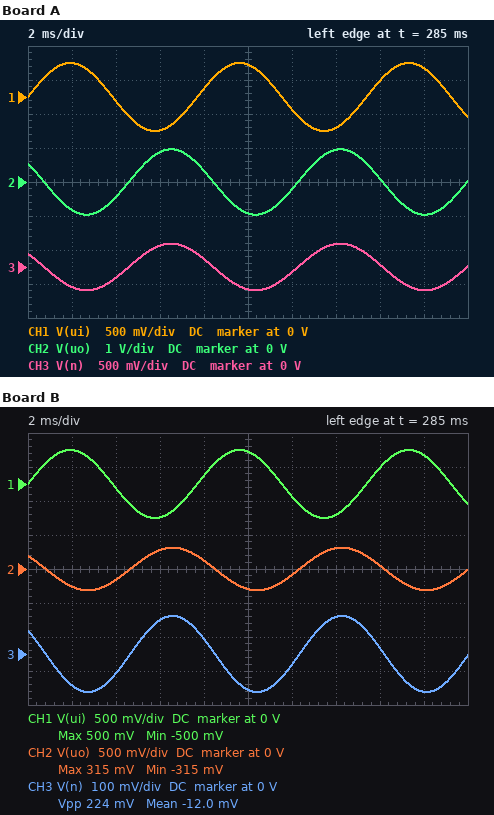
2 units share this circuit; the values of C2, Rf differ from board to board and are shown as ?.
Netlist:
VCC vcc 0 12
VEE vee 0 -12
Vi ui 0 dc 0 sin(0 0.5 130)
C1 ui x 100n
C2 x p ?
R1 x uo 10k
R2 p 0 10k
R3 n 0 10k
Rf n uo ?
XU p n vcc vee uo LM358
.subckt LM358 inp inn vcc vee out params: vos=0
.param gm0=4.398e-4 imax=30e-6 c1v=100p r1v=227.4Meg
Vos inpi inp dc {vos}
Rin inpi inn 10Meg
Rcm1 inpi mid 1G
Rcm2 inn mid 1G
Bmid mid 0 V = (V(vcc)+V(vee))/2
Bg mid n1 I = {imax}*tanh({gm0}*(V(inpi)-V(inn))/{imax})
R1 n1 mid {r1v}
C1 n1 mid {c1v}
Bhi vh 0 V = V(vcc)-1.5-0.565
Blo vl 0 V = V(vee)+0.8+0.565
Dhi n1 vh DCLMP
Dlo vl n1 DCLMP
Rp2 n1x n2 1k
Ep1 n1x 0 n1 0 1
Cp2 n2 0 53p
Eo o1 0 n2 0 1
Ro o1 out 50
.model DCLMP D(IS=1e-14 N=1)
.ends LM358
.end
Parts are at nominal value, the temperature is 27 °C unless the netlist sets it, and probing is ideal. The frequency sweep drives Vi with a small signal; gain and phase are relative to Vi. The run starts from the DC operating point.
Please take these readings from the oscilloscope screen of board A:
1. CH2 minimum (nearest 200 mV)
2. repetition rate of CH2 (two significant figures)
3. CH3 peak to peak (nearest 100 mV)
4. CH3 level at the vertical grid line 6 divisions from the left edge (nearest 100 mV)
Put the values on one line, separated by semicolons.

-1.0 V; 130 Hz; 700 mV; -100 mV
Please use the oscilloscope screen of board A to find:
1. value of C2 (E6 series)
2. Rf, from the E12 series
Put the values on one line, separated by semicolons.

68 nF; 18 kΩ
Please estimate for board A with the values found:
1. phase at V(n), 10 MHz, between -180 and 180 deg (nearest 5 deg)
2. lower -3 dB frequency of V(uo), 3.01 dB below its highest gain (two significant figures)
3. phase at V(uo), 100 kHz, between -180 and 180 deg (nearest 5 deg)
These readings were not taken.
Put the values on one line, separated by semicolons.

-155 deg; 160 Hz; -20 deg
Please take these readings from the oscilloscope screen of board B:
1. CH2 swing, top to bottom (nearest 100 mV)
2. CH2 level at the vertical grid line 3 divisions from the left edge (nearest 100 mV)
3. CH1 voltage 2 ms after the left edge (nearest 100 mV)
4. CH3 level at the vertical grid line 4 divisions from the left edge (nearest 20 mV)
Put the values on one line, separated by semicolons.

600 mV; 300 mV; 500 mV; 40 mV
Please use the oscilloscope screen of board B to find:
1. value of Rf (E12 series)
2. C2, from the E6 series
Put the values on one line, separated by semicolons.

18 kΩ; 33 nF
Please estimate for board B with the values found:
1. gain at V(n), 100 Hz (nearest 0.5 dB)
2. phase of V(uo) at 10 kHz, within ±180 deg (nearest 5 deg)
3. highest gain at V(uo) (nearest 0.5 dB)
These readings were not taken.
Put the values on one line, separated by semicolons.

-17.5 dB; 0 deg; 9.0 dB
